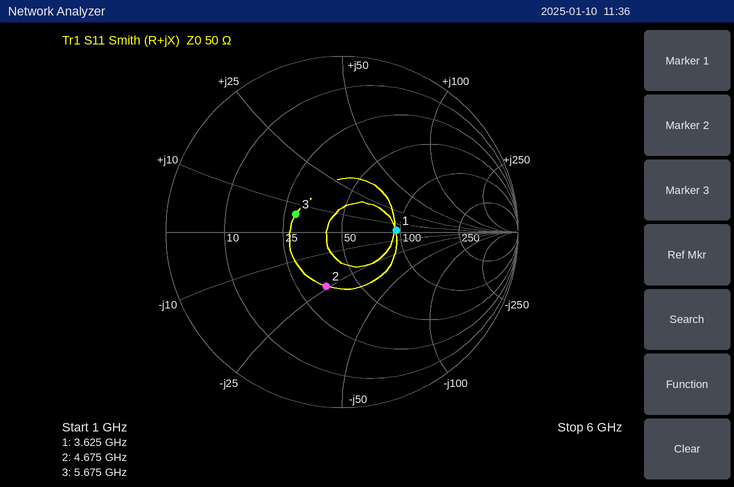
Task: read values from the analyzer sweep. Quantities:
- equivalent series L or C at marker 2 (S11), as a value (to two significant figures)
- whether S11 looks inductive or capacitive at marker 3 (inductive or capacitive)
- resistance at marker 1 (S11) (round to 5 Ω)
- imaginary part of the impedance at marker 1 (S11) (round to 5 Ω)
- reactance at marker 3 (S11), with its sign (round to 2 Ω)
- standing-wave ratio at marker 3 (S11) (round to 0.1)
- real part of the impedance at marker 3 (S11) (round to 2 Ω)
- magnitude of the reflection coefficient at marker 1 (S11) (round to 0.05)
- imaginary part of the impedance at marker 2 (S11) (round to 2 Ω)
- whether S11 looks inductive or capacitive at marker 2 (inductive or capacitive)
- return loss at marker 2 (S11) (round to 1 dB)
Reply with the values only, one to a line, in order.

1.4 pF
inductive
95 Ω
0 Ω
+6 Ω
1.8
28 Ω
0.30
-24 Ω
capacitive
10 dB
